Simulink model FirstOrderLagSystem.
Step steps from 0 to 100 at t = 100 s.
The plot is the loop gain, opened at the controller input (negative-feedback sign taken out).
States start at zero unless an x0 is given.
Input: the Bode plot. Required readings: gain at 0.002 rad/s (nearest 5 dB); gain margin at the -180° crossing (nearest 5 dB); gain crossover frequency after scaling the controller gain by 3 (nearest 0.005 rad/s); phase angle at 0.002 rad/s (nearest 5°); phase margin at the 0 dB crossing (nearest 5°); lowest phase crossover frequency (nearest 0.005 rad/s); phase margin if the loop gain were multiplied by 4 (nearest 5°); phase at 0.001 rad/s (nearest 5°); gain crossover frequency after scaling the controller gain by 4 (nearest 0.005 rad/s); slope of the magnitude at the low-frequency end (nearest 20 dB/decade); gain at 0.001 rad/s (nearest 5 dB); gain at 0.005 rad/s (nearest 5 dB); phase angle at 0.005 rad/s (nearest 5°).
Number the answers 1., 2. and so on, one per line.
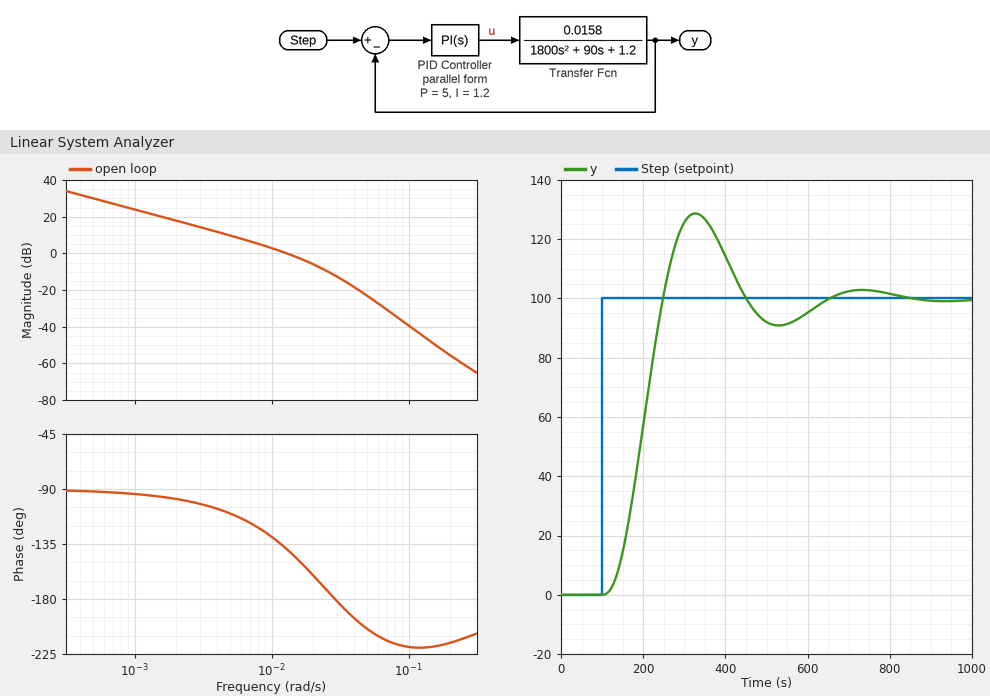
1. 20 dB
2. 10 dB
3. 0.025 rad/s
4. -100°
5. 40°
6. 0.030 rad/s
7. 0°
8. -95°
9. 0.030 rad/s
10. -20 dB/decade
11. 25 dB
12. 10 dB
13. -110°
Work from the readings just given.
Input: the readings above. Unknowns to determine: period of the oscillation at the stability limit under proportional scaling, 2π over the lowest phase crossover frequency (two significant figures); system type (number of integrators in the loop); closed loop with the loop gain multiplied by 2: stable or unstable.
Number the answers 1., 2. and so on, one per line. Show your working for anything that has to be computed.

1. 2π / 0.03 = 210 s
2. 1
3. stable
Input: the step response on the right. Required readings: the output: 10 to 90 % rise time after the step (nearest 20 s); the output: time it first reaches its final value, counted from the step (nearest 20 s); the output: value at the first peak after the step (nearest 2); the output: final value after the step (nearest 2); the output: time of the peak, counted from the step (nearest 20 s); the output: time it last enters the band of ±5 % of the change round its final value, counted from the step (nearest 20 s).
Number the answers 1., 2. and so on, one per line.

1. 100 s
2. 140 s
3. 128
4. 100
5. 220 s
6. 500 s
